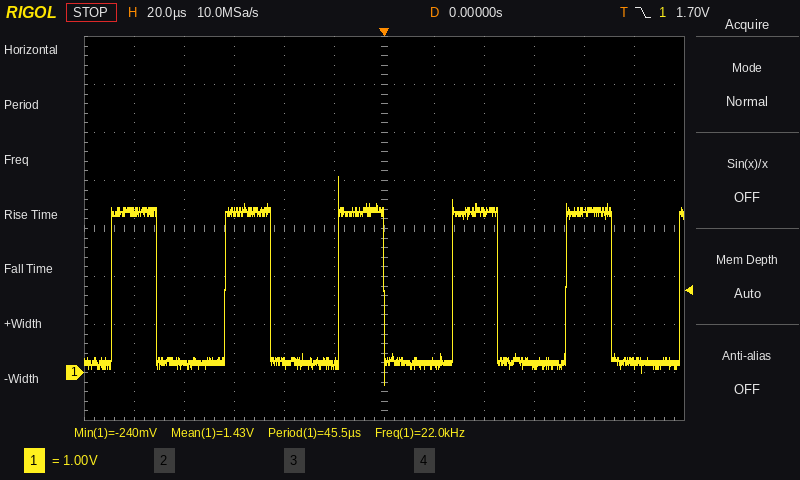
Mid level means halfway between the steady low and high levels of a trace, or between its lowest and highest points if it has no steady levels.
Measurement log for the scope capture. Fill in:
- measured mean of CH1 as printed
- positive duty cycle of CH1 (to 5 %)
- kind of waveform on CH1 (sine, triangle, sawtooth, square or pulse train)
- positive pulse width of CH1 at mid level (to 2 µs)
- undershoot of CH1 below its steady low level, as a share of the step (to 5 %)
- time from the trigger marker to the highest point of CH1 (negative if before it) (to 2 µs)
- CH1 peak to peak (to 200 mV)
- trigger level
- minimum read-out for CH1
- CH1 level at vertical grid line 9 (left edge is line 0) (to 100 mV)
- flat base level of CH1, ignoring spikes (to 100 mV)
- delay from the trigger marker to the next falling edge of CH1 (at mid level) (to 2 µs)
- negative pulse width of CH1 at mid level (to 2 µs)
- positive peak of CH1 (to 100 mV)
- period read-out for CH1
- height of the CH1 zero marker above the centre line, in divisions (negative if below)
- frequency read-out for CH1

1.43 V
40 %
pulse train
18 µs
15 %
-18 µs
4.4 V
1.70 V
-240 mV
200 mV
200 mV
46 µs
28 µs
4.1 V
45.5 µs
-3.0 div
22.0 kHz
